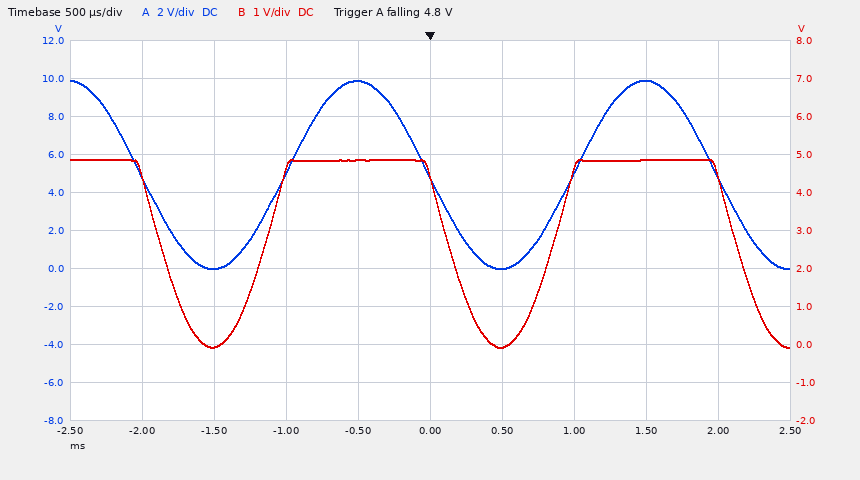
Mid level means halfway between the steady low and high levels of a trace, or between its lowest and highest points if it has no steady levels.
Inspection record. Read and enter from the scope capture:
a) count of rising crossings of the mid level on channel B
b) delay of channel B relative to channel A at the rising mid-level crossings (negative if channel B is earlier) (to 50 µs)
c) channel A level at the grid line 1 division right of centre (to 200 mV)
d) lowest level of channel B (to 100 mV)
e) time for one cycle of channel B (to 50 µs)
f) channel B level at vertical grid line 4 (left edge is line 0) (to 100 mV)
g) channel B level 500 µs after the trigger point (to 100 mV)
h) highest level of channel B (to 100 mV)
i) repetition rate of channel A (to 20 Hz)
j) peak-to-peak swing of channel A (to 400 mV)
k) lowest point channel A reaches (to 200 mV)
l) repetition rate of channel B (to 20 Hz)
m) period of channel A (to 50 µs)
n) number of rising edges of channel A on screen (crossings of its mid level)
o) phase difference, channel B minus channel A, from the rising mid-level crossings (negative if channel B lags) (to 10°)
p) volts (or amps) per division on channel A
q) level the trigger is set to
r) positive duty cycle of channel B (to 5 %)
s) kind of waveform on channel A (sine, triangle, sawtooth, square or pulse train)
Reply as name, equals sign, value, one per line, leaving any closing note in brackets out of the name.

count of rising crossings of the mid level on channel B = 2
delay of channel B relative to channel A at the rising mid-level crossings (negative if channel B is earlier) = -150 µs
channel A level at the grid line 1 division right of centre = 0.0 V
lowest level of channel B = -100 mV
time for one cycle of channel B = 2.00 ms
channel B level at vertical grid line 4 (left edge is line 0) = 4.9 V
channel B level 500 µs after the trigger point = -100 mV
highest level of channel B = 4.9 V
repetition rate of channel A = 500 Hz
peak-to-peak swing of channel A = 10.0 V
lowest point channel A reaches = 0.0 V
repetition rate of channel B = 500 Hz
period of channel A = 2.00 ms
number of rising edges of channel A on screen = 2
phase difference, channel B minus channel A, from the rising mid-level crossings (negative if channel B lags) = +30°
volts (or amps) per division on channel A = 2 V
level the trigger is set to = 4.8 V
positive duty cycle of channel B = 65 %
kind of waveform on channel A = sine
